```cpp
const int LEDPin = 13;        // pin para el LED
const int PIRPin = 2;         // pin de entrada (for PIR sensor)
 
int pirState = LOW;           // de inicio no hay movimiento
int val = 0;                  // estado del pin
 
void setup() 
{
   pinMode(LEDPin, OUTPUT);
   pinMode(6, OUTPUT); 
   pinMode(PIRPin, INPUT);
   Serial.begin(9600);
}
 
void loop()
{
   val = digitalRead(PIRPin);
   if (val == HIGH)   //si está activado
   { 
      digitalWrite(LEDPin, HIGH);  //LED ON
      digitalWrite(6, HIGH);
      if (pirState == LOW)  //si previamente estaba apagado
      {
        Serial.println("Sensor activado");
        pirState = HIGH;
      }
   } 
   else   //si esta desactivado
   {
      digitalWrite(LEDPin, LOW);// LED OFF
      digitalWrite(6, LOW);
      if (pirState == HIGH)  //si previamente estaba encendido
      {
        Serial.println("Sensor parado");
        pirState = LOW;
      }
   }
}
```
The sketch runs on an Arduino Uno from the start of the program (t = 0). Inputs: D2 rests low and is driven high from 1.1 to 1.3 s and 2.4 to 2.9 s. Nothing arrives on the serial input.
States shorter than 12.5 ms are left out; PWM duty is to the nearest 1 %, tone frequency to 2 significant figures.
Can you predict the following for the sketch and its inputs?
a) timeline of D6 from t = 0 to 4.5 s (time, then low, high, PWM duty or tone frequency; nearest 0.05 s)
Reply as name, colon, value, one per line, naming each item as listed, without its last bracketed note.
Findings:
timeline of D6 from t = 0 to 4.5 s: 0 s low; 1.1 s high; 1.3 s low; 2.4 s high; 2.9 s low
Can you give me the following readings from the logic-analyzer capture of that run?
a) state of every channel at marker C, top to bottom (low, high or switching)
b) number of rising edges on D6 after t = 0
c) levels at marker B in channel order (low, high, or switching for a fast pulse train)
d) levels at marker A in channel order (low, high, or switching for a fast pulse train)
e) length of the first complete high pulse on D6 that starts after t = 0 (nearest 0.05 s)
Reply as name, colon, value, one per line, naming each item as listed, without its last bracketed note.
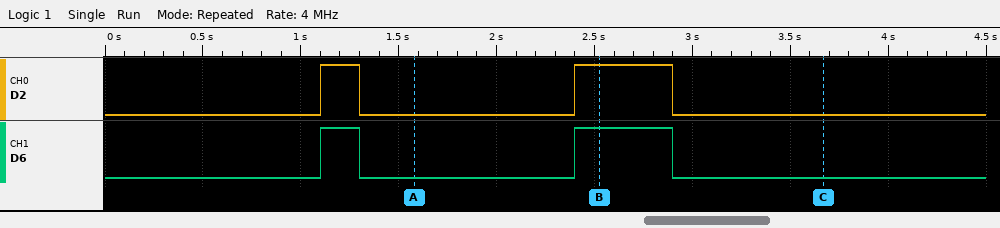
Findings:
state of every channel at marker C, top to bottom: D2 low, D6 low
number of rising edges on D6 after t = 0: 2
levels at marker B in channel order: D2 high, D6 high
levels at marker A in channel order: D2 low, D6 low
length of the first complete high pulse on D6 that starts after t = 0: 0.20 s
